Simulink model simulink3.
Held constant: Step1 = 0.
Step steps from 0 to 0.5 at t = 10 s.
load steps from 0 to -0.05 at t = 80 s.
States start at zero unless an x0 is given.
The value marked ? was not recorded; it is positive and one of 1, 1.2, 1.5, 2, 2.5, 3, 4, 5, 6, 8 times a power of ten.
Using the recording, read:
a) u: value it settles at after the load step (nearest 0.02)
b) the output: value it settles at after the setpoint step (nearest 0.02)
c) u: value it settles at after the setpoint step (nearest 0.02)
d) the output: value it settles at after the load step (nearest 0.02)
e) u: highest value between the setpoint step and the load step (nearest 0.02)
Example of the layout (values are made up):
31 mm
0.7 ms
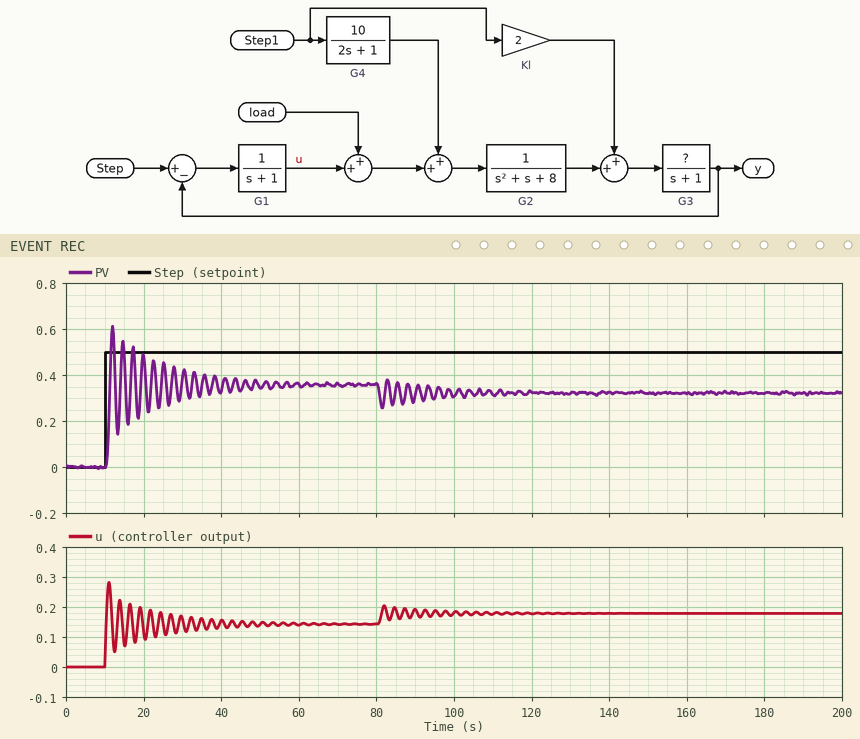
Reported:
0.18
0.36
0.14
0.32
0.28
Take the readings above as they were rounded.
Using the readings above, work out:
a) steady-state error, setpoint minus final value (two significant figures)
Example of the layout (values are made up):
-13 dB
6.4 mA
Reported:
0.14
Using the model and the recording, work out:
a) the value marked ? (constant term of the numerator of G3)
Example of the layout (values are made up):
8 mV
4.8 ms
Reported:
20
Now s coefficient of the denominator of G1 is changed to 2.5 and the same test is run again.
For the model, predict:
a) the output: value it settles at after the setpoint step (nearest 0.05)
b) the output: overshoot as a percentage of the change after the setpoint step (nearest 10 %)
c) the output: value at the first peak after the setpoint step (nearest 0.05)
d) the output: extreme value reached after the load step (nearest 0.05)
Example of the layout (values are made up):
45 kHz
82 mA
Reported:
0.35
20 %
0.45
0.25
